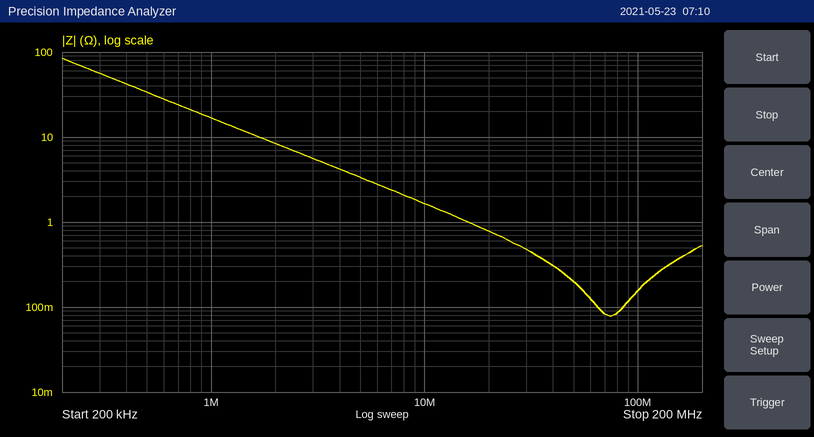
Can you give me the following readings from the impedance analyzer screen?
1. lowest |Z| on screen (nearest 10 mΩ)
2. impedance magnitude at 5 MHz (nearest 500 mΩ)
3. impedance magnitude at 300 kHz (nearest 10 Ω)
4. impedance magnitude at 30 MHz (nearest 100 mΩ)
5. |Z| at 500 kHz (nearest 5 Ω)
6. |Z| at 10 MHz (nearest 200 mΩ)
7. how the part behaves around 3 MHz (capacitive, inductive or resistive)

80 mΩ
3.5 Ω
60 Ω
500 mΩ
35 Ω
1.6 Ω
capacitive
